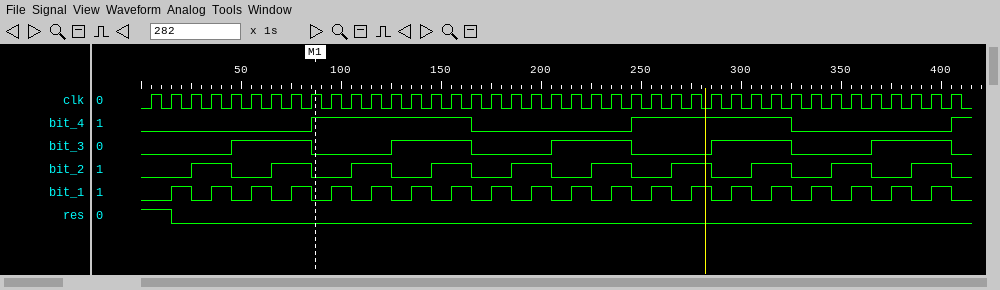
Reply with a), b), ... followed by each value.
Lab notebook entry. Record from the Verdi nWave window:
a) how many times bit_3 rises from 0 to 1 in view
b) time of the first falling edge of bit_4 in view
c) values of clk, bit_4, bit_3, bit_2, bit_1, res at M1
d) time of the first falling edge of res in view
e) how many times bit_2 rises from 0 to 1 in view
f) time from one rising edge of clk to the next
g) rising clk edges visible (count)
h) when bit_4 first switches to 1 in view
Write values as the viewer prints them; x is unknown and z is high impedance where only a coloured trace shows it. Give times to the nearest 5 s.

a) 5
b) 165 s
c) clk=1, bit_4=1, bit_3=0, bit_2=0, bit_1=0, res=0
d) 15 s
e) 10
f) 10 s
g) 41
h) 85 s
